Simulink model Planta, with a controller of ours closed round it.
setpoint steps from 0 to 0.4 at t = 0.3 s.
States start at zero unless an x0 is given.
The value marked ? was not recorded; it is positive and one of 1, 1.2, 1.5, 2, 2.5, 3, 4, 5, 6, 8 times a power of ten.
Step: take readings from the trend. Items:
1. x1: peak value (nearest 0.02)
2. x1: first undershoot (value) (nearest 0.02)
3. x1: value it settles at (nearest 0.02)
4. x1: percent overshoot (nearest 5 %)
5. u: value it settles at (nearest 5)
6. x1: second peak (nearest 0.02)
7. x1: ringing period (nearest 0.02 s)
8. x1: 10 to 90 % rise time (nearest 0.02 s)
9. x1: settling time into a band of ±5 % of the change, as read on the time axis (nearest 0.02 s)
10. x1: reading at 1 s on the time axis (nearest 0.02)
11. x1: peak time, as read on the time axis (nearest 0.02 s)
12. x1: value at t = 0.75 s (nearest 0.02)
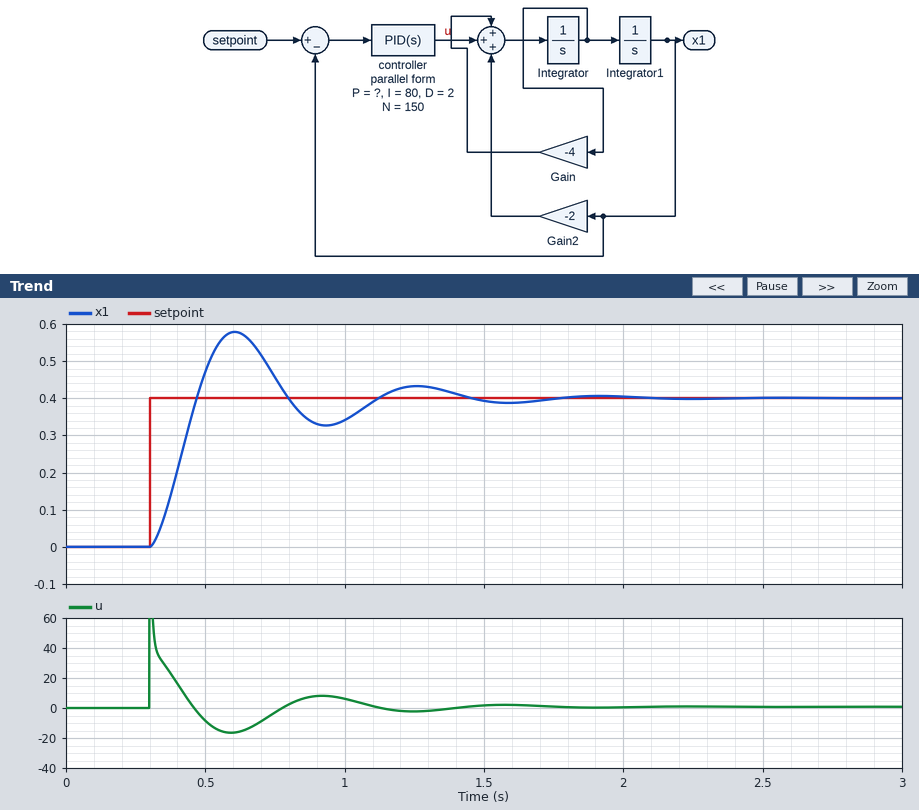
0.58
0.32
0.40
45 %
0
0.44
0.66 s
0.12 s
1.36 s
0.34
0.60 s
0.46
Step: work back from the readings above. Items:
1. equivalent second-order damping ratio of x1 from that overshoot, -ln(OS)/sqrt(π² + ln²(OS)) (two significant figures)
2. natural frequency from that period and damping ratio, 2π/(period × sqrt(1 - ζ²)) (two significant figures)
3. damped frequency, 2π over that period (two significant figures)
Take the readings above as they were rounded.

0.25
9.8 rad/s
9.5 rad/s
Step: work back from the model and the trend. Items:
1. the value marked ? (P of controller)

100
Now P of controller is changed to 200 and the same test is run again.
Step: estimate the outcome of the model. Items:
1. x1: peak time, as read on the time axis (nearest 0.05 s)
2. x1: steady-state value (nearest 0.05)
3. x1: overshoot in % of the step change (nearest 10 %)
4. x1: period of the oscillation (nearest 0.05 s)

0.50 s
0.40
50 %
0.45 s
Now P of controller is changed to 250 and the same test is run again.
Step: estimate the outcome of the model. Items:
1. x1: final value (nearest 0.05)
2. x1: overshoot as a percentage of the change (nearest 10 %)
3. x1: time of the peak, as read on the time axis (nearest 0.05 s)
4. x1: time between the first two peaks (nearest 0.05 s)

0.40
60 %
0.50 s
0.40 s
